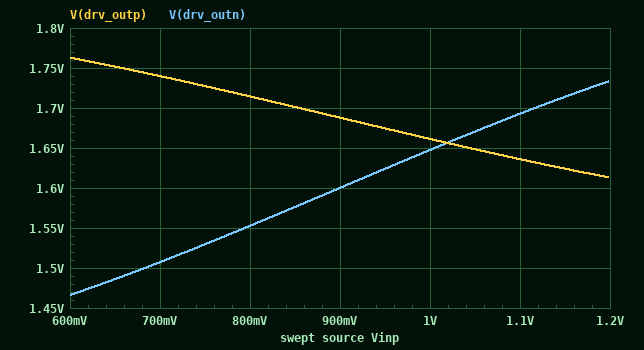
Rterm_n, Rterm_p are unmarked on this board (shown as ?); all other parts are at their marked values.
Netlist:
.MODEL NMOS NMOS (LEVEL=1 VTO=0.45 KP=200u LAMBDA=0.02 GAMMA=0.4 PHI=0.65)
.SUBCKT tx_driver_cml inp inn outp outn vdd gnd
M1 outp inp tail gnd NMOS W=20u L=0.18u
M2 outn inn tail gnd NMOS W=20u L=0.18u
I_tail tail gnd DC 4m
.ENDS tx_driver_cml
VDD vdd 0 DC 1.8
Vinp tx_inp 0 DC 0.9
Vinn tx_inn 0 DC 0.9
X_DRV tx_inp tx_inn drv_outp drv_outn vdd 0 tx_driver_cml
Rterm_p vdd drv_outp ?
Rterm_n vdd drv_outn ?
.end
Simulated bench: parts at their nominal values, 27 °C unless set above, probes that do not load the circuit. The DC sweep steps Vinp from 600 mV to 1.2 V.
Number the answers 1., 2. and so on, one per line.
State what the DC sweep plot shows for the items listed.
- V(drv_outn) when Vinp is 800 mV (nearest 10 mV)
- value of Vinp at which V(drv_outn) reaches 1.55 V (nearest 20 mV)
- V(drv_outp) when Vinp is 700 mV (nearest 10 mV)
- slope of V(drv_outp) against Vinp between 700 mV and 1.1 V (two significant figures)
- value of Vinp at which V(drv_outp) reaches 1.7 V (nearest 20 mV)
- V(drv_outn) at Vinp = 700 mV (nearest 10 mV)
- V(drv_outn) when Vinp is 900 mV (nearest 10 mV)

1. 1.55 V
2. 800 mV
3. 1.74 V
4. -0.26 V/V
5. 860 mV
6. 1.51 V
7. 1.60 V
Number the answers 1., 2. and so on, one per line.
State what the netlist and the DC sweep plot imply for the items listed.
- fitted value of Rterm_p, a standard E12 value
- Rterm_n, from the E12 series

1. 56 Ω
2. 100 Ω
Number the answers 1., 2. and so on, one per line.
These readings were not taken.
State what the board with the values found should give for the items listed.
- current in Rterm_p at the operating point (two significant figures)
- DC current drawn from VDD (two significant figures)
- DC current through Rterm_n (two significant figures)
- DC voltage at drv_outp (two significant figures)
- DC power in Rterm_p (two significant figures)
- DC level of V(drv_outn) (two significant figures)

1. 2.0 mA
2. 4.0 mA
3. 2.0 mA
4. 1.7 V
5. 220 µW
6. 1.6 V
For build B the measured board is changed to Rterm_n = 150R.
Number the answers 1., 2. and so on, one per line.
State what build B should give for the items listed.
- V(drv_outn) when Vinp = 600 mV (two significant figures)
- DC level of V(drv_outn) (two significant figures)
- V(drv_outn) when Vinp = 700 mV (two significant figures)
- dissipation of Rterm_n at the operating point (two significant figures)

1. 1.3 V
2. 1.5 V
3. 1.4 V
4. 600 µW
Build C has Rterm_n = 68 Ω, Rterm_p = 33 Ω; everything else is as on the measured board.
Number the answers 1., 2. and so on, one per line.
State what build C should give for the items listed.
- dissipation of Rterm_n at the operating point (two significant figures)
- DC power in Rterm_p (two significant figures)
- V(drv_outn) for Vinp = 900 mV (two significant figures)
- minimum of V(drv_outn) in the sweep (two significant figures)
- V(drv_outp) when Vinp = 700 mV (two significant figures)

1. 270 µW
2. 130 µW
3. 1.7 V
4. 1.6 V
5. 1.8 V
